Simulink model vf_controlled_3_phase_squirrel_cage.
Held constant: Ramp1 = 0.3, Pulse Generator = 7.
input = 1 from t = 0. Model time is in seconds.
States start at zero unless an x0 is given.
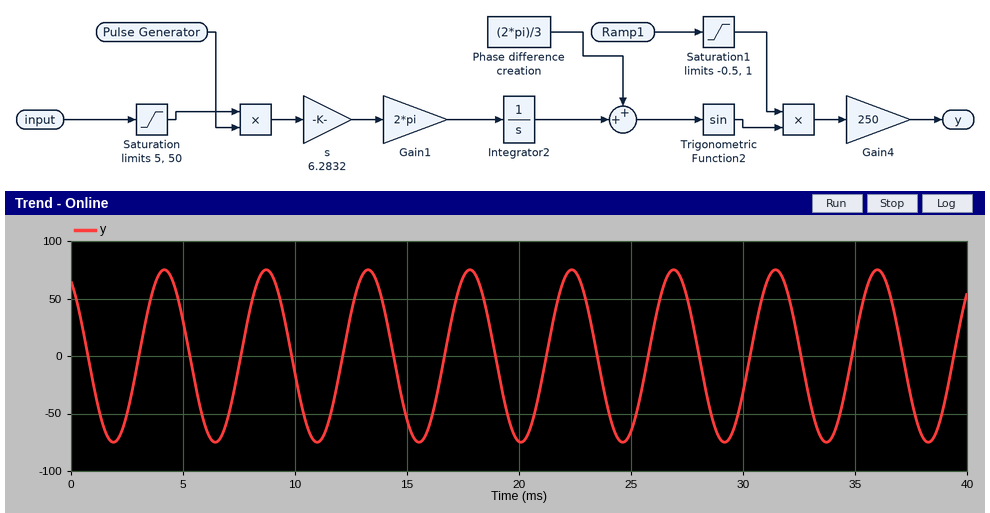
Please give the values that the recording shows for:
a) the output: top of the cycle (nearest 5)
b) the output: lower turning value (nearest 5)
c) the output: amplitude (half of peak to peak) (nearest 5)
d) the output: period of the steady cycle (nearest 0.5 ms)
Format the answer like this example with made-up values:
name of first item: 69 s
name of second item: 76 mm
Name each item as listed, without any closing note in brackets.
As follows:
the output: top of the cycle: 75
the output: lower turning value: -75
the output: amplitude (half of peak to peak): 75
the output: period of the steady cycle: 4.5 ms
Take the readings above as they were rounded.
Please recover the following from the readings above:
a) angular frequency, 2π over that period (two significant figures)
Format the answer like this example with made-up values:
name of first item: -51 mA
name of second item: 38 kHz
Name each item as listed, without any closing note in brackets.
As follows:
angular frequency, 2π over that period: 1.4 rad/ms
